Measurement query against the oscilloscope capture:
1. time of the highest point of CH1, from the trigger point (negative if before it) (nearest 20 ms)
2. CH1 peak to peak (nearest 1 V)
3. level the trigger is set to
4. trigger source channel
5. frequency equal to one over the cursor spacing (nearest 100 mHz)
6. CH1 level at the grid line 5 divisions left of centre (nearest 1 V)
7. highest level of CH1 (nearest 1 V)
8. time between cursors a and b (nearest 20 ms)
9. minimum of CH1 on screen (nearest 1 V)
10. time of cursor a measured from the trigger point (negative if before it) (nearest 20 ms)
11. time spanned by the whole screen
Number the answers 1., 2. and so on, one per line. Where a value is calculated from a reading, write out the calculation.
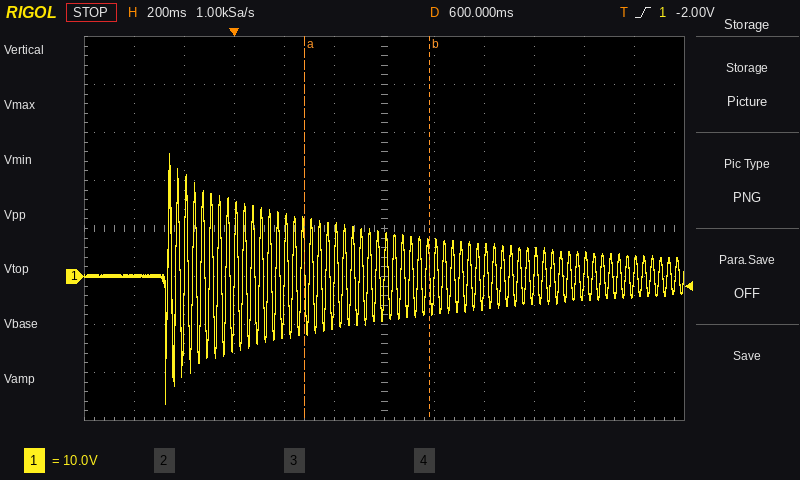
1. -260 ms
2. 26 V − (-26 V) = 52 V
3. -2.00 V
4. CH1
5. 1 / 500 ms ≈ 2.0 Hz
6. 0 V
7. 26 V
8. 500 ms
9. -26 V
10. +280 ms
11. 2.4 s
